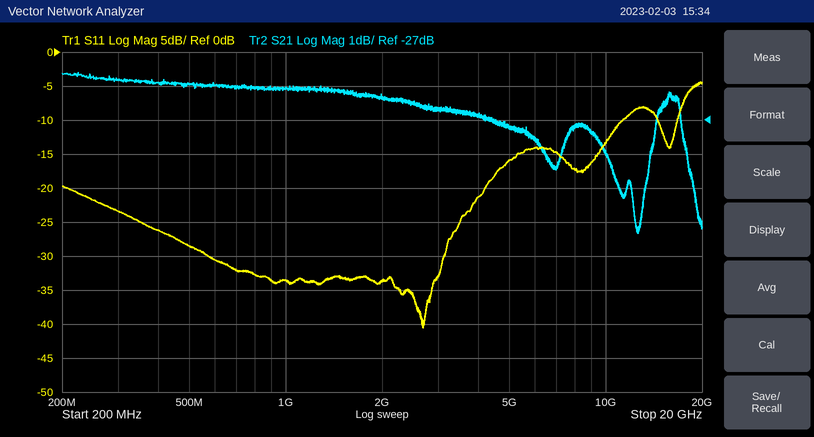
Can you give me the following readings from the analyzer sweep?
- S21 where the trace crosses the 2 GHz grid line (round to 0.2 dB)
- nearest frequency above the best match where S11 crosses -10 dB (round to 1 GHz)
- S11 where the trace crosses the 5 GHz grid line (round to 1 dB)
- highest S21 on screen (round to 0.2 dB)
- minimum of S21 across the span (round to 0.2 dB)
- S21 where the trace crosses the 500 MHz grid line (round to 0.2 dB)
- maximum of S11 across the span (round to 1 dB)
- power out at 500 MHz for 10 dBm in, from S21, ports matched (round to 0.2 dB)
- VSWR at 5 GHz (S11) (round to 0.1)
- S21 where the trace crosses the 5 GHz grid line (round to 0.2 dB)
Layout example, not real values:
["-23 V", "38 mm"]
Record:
["-26.4 dB", "11 GHz", "-16 dB", "-25.6 dB", "-30.4 dB", "-26.0 dB", "-4 dB", "-16.0 dBm", "1.4", "-27.2 dB"]
